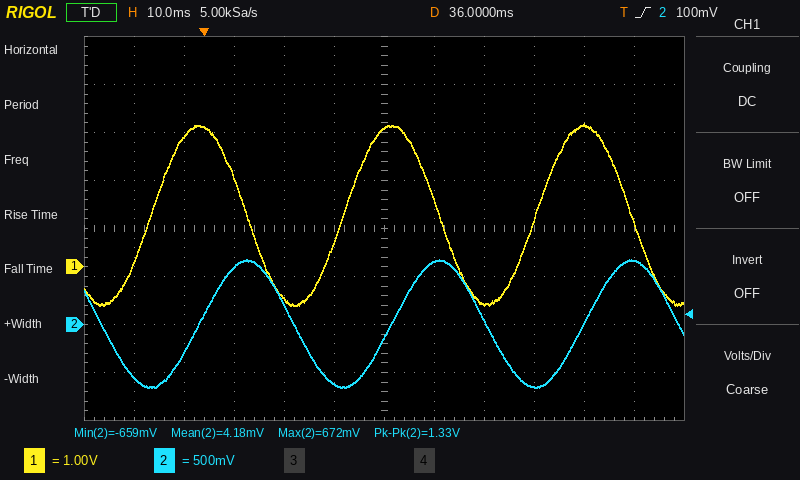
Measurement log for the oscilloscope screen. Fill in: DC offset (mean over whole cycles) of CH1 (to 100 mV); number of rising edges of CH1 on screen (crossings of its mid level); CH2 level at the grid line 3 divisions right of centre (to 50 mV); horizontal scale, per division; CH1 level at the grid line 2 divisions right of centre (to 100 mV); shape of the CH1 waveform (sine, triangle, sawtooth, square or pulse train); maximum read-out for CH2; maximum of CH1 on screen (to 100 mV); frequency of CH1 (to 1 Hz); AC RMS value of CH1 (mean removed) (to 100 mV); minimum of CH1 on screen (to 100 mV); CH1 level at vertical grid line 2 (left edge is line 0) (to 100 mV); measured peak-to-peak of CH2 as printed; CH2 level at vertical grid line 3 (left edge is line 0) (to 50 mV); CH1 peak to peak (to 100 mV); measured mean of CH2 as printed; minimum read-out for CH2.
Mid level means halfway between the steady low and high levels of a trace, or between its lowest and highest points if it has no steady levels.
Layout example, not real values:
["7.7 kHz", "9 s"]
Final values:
["1.1 V", "3", "-650 mV", "10 ms", "-800 mV", "sine", "672 mV", "3.0 V", "26 Hz", "1.3 V", "-800 mV", "2.7 V", "1.33 V", "600 mV", "3.8 V", "4.18 mV", "-659 mV"]
